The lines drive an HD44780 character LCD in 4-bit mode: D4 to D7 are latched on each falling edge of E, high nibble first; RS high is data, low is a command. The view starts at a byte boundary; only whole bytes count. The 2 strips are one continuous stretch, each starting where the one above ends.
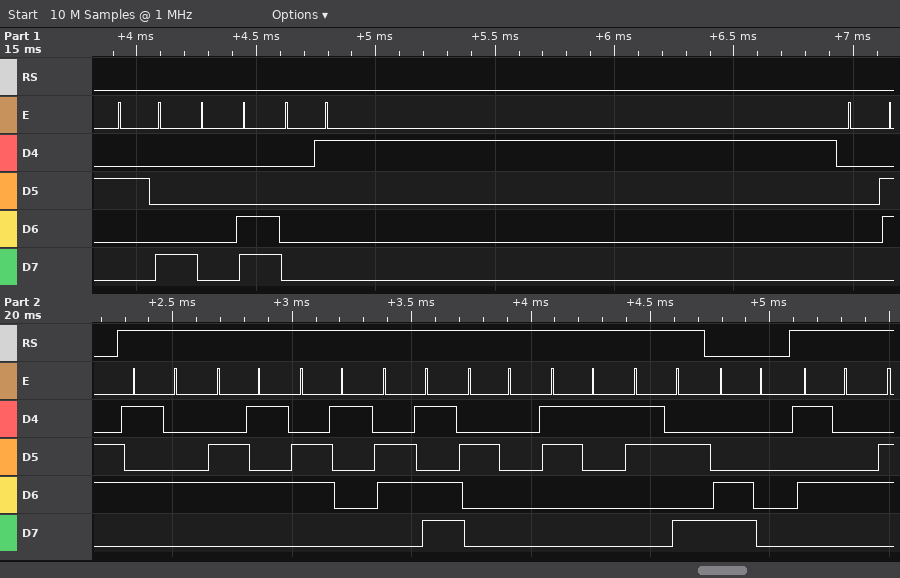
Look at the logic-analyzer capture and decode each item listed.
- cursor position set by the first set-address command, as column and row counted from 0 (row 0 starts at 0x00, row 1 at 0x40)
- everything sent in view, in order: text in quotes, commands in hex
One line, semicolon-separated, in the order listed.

column 0, row 1; 0x28 0x0C 0x01 0x06 "Team 1:" 0xC0 "T"
